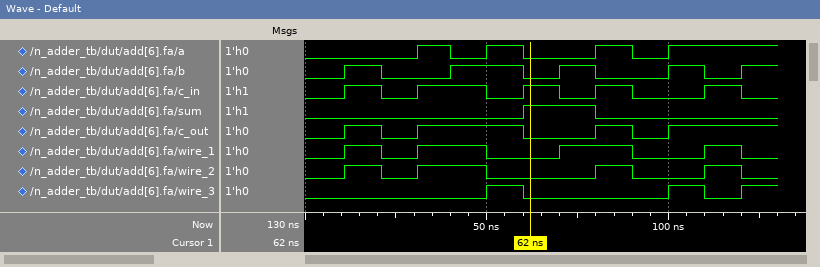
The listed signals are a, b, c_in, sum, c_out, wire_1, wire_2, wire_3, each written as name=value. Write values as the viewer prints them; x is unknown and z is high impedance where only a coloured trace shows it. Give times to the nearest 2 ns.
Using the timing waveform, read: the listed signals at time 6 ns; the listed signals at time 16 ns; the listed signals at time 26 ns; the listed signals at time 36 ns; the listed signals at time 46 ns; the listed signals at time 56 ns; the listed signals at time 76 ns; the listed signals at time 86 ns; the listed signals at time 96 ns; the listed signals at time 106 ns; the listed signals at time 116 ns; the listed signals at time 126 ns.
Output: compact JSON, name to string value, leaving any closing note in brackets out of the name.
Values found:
{"the listed signals at time 6 ns": "a=0, b=0, c_in=0, sum=0, c_out=0, wire_1=0, wire_2=0, wire_3=0", "the listed signals at time 16 ns": "a=0, b=1, c_in=1, sum=0, c_out=1, wire_1=1, wire_2=1, wire_3=0", "the listed signals at time 26 ns": "a=0, b=0, c_in=0, sum=0, c_out=0, wire_1=0, wire_2=0, wire_3=0", "the listed signals at time 36 ns": "a=1, b=0, c_in=1, sum=0, c_out=1, wire_1=1, wire_2=1, wire_3=0", "the listed signals at time 46 ns": "a=0, b=1, c_in=1, sum=0, c_out=1, wire_1=1, wire_2=1, wire_3=0", "the listed signals at time 56 ns": "a=1, b=1, c_in=0, sum=0, c_out=1, wire_1=0, wire_2=0, wire_3=1", "the listed signals at time 76 ns": "a=0, b=1, c_in=0, sum=1, c_out=0, wire_1=1, wire_2=0, wire_3=0", "the listed signals at time 86 ns": "a=1, b=0, c_in=1, sum=0, c_out=1, wire_1=1, wire_2=1, wire_3=0", "the listed signals at time 96 ns": "a=0, b=0, c_in=0, sum=0, c_out=0, wire_1=0, wire_2=0, wire_3=0", "the listed signals at time 106 ns": "a=1, b=1, c_in=0, sum=0, c_out=1, wire_1=0, wire_2=0, wire_3=1", "the listed signals at time 116 ns": "a=1, b=0, c_in=1, sum=0, c_out=1, wire_1=1, wire_2=1, wire_3=0", "the listed signals at time 126 ns": "a=1, b=1, c_in=0, sum=0, c_out=1, wire_1=0, wire_2=0, wire_3=1"}
